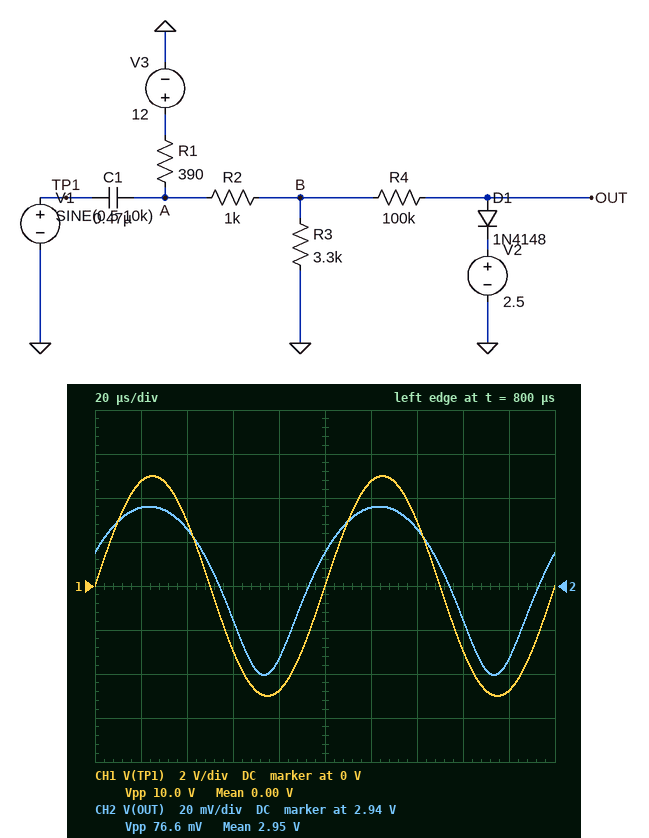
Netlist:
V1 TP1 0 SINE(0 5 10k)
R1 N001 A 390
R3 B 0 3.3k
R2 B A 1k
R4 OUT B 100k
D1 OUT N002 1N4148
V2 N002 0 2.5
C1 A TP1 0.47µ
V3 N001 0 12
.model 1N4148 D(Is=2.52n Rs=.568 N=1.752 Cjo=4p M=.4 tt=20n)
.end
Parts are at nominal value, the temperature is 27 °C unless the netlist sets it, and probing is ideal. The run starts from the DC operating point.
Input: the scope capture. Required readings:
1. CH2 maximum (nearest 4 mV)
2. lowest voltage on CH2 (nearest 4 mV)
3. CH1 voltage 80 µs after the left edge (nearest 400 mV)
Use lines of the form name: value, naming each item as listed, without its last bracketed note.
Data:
CH2 maximum: 2.976 V
lowest voltage on CH2: 2.900 V
CH1 voltage 80 µs after the left edge: -4.8 V
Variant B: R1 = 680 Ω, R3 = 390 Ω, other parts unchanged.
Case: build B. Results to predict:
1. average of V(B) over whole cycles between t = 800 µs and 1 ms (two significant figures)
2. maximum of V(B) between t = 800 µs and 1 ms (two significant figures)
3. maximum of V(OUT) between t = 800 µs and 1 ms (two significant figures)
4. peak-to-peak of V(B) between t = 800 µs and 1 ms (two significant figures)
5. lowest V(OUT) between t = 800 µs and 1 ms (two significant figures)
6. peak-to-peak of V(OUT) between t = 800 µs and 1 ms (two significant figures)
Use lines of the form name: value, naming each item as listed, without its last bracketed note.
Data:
average of V(B) over whole cycles between t = 800 µs and 1 ms: 2.3 V
maximum of V(B) between t = 800 µs and 1 ms: 3.7 V
maximum of V(OUT) between t = 800 µs and 1 ms: 2.9 V
peak-to-peak of V(B) between t = 800 µs and 1 ms: 2.8 V
lowest V(OUT) between t = 800 µs and 1 ms: 860 mV
peak-to-peak of V(OUT) between t = 800 µs and 1 ms: 2.0 V
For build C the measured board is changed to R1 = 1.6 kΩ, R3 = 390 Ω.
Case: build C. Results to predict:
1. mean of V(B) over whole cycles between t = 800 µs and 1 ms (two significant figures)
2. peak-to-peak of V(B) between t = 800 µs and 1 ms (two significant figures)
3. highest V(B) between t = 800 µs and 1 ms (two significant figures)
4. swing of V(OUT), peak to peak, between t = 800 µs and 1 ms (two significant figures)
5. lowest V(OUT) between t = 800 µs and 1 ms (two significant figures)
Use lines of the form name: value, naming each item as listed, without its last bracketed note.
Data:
mean of V(B) over whole cycles between t = 800 µs and 1 ms: 1.6 V
peak-to-peak of V(B) between t = 800 µs and 1 ms: 2.8 V
highest V(B) between t = 800 µs and 1 ms: 3.0 V
swing of V(OUT), peak to peak, between t = 800 µs and 1 ms: 2.6 V
lowest V(OUT) between t = 800 µs and 1 ms: 160 mV
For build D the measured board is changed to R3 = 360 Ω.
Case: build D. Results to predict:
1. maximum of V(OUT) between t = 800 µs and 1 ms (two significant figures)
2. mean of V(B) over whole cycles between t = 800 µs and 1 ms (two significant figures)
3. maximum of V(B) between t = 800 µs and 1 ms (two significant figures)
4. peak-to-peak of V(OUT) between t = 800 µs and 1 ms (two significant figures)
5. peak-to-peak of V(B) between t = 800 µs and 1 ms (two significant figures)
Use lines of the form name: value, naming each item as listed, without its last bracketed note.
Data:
maximum of V(OUT) between t = 800 µs and 1 ms: 2.9 V
mean of V(B) over whole cycles between t = 800 µs and 1 ms: 2.5 V
maximum of V(B) between t = 800 µs and 1 ms: 3.8 V
peak-to-peak of V(OUT) between t = 800 µs and 1 ms: 1.7 V
peak-to-peak of V(B) between t = 800 µs and 1 ms: 2.6 V
